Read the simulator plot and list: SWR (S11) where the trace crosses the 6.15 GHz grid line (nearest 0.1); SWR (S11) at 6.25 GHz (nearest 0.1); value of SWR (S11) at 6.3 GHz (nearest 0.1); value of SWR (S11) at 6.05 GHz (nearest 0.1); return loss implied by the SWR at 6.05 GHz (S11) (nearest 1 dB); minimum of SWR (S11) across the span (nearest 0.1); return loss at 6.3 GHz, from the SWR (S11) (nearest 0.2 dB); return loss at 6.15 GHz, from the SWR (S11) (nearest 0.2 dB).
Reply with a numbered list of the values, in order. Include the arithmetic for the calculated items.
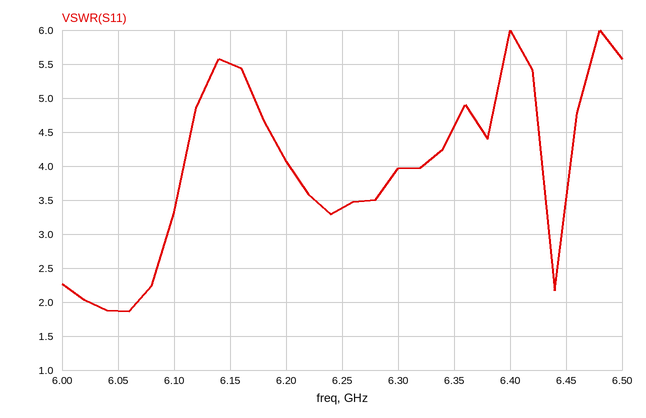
1. 5.5
2. 3.4
3. 4.0
4. 1.9
5. −20 log10((1.9 − 1)/(1.9 + 1)) ≈ 10 dB
6. 1.9
7. −20 log10((4 − 1)/(4 + 1)) ≈ 4.4 dB
8. −20 log10((5.5 − 1)/(5.5 + 1)) ≈ 3.2 dB
